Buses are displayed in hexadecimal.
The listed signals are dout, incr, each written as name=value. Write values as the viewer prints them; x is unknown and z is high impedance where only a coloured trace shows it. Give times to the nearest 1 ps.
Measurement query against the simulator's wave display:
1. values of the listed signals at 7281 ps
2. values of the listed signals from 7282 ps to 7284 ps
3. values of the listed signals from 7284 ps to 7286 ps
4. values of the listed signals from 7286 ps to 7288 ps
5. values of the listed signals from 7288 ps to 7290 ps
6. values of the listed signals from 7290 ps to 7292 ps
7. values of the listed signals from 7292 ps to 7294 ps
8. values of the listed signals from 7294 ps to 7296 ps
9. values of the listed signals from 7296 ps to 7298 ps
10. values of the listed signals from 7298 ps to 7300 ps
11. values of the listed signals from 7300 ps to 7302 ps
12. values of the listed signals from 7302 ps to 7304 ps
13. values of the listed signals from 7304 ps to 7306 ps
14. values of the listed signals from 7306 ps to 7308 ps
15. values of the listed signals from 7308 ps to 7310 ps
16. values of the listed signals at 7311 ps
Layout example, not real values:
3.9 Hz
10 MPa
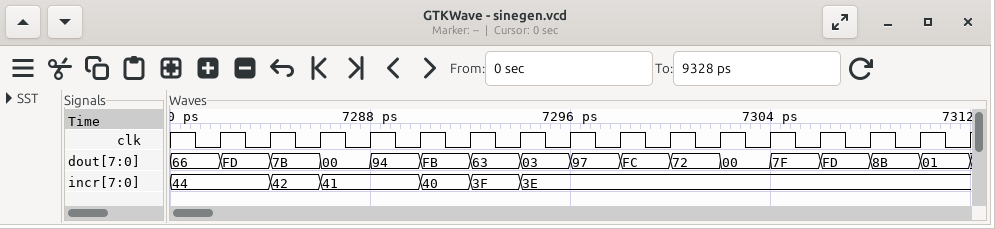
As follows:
dout=66, incr=44
dout=FD, incr=44
dout=7B, incr=42
dout=00, incr=41
dout=94, incr=41
dout=FB, incr=40
dout=63, incr=3F
dout=03, incr=3E
dout=97, incr=3E
dout=FC, incr=3E
dout=72, incr=3E
dout=00, incr=3E
dout=7F, incr=3E
dout=FD, incr=3E
dout=8B, incr=3E
dout=01, incr=3E
